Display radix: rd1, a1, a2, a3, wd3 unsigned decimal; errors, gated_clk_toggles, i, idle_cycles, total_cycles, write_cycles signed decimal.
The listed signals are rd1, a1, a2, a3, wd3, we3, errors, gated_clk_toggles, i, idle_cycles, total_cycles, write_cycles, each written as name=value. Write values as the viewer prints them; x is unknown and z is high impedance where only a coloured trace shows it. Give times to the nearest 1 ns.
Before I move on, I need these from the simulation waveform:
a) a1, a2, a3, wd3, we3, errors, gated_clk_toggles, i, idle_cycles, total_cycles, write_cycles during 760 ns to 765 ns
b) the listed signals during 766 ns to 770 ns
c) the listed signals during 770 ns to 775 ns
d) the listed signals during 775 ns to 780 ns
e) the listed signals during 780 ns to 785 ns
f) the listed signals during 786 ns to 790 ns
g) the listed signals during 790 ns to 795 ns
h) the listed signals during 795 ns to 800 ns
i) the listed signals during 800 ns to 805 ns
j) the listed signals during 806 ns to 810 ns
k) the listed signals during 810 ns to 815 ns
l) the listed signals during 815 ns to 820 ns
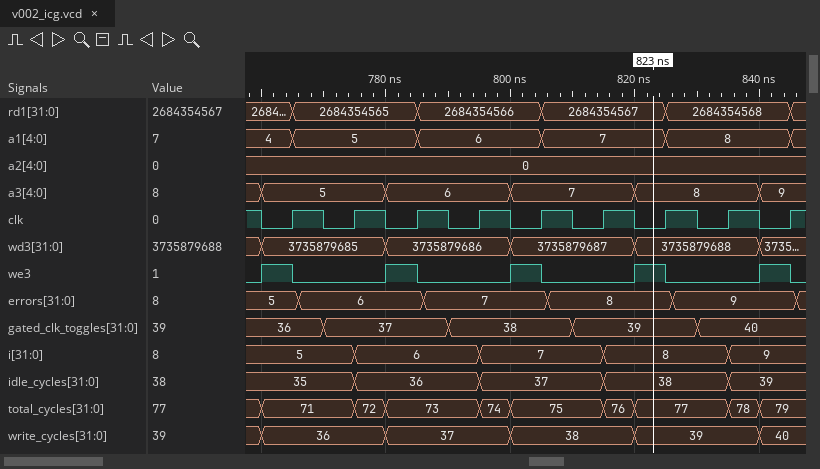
a1=4, a2=0, a3=5, wd3=3735879685, we3=1, errors=5, gated_clk_toggles=36, i=5, idle_cycles=35, total_cycles=71, write_cycles=36
rd1=2684354565, a1=5, a2=0, a3=5, wd3=3735879685, we3=0, errors=6, gated_clk_toggles=36, i=5, idle_cycles=35, total_cycles=71, write_cycles=36
rd1=2684354565, a1=5, a2=0, a3=5, wd3=3735879685, we3=0, errors=6, gated_clk_toggles=37, i=5, idle_cycles=35, total_cycles=71, write_cycles=36
rd1=2684354565, a1=5, a2=0, a3=5, wd3=3735879685, we3=0, errors=6, gated_clk_toggles=37, i=6, idle_cycles=36, total_cycles=72, write_cycles=36
rd1=2684354565, a1=5, a2=0, a3=6, wd3=3735879686, we3=1, errors=6, gated_clk_toggles=37, i=6, idle_cycles=36, total_cycles=73, write_cycles=37
rd1=2684354566, a1=6, a2=0, a3=6, wd3=3735879686, we3=0, errors=7, gated_clk_toggles=37, i=6, idle_cycles=36, total_cycles=73, write_cycles=37
rd1=2684354566, a1=6, a2=0, a3=6, wd3=3735879686, we3=0, errors=7, gated_clk_toggles=38, i=6, idle_cycles=36, total_cycles=73, write_cycles=37
rd1=2684354566, a1=6, a2=0, a3=6, wd3=3735879686, we3=0, errors=7, gated_clk_toggles=38, i=7, idle_cycles=37, total_cycles=74, write_cycles=37
rd1=2684354566, a1=6, a2=0, a3=7, wd3=3735879687, we3=1, errors=7, gated_clk_toggles=38, i=7, idle_cycles=37, total_cycles=75, write_cycles=38
rd1=2684354567, a1=7, a2=0, a3=7, wd3=3735879687, we3=0, errors=8, gated_clk_toggles=38, i=7, idle_cycles=37, total_cycles=75, write_cycles=38
rd1=2684354567, a1=7, a2=0, a3=7, wd3=3735879687, we3=0, errors=8, gated_clk_toggles=39, i=7, idle_cycles=37, total_cycles=75, write_cycles=38
rd1=2684354567, a1=7, a2=0, a3=7, wd3=3735879687, we3=0, errors=8, gated_clk_toggles=39, i=8, idle_cycles=38, total_cycles=76, write_cycles=38
